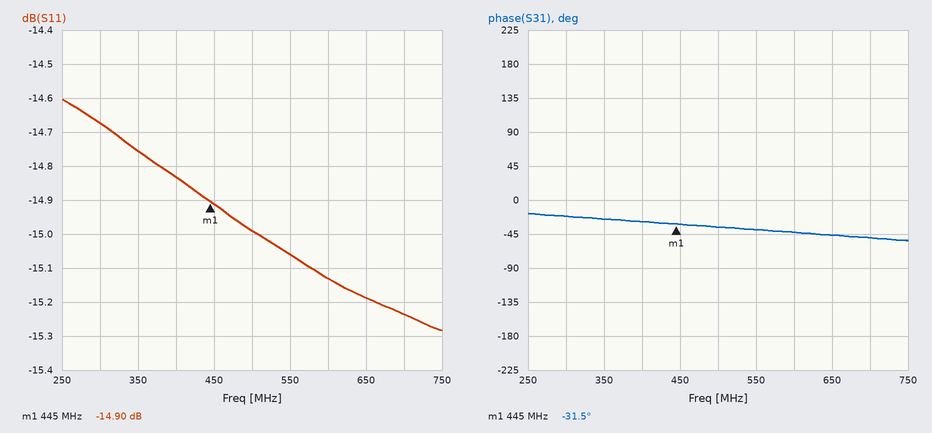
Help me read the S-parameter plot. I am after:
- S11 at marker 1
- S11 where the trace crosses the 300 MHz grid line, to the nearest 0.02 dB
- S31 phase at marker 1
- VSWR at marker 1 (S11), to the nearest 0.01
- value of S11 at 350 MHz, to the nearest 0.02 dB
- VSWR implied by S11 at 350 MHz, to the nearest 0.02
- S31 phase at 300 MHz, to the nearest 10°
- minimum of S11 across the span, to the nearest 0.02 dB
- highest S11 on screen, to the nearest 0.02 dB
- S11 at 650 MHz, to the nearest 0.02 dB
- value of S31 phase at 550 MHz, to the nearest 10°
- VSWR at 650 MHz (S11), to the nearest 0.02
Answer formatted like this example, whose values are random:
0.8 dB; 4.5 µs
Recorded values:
-14.90 dB; -14.68 dB; -31.5°; 1.44; -14.76 dB; 1.44; -20°; -15.28 dB; -14.60 dB; -15.18 dB; -40°; 1.42
